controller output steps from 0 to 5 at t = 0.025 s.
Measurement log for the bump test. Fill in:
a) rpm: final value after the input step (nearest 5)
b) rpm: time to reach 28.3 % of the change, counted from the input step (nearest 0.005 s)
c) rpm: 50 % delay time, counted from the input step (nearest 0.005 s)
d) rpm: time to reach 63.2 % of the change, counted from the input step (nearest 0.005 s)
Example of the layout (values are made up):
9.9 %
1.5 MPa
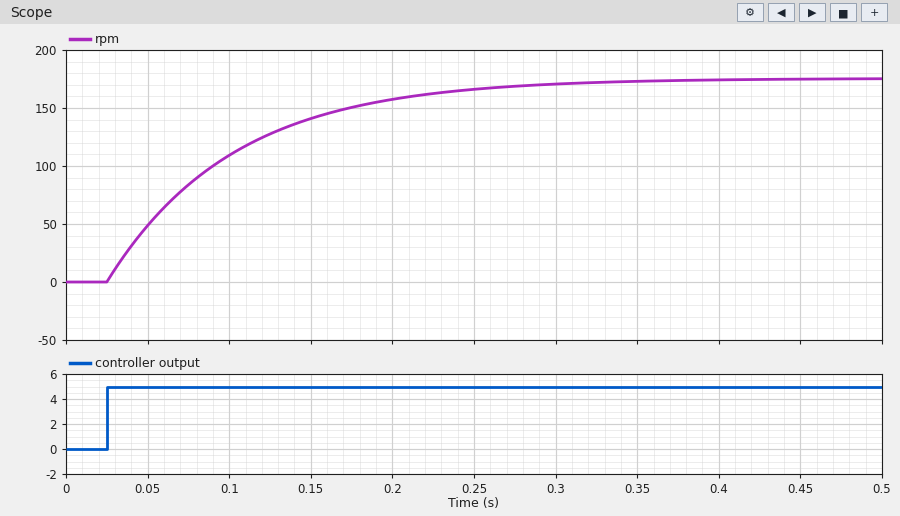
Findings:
175
0.025 s
0.055 s
0.075 s
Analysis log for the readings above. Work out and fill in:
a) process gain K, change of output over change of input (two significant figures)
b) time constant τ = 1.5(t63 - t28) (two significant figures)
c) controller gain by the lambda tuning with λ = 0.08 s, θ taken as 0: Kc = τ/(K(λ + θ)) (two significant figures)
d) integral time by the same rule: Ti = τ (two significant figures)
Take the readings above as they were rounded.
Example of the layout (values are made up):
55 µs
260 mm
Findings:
35
0.075 s
0.027
0.075 s
